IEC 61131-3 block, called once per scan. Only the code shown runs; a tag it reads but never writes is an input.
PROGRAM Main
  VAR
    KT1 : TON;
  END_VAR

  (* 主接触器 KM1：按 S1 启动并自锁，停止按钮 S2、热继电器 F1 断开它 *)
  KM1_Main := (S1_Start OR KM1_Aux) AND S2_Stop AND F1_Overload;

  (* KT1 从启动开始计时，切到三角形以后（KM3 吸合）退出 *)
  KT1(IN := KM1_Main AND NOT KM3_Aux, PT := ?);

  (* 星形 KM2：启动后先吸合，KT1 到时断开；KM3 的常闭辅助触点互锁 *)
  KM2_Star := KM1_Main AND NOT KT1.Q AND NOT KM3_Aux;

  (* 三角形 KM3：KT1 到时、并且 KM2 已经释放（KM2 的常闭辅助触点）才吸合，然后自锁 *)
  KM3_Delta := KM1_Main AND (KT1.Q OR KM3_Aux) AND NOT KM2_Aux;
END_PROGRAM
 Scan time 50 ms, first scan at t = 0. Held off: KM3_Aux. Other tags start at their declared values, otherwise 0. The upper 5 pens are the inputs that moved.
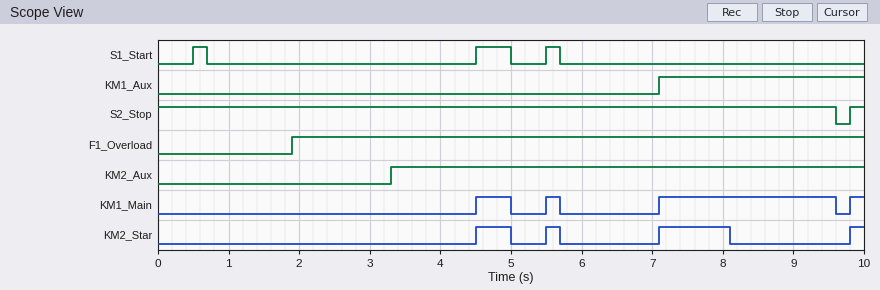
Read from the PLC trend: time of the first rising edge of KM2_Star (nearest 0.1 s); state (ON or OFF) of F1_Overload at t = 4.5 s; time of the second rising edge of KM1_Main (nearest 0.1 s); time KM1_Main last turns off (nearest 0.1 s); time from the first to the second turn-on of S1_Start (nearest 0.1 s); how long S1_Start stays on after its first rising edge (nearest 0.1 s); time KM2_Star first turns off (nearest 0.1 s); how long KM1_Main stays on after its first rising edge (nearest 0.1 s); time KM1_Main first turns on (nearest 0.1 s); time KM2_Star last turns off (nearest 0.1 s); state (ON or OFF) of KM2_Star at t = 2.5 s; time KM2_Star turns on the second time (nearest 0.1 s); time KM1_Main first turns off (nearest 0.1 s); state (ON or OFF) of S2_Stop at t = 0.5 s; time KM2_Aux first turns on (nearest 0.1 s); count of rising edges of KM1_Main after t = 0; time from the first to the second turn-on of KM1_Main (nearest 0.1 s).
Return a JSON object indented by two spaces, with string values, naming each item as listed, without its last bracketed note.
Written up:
{
  "time of the first rising edge of KM2_Star": "4.5 s",
  "state (ON or OFF) of F1_Overload at t = 4.5 s": "ON",
  "time of the second rising edge of KM1_Main": "5.5 s",
  "time KM1_Main last turns off": "9.6 s",
  "time from the first to the second turn-on of S1_Start": "4.0 s",
  "how long S1_Start stays on after its first rising edge": "0.2 s",
  "time KM2_Star first turns off": "5.0 s",
  "how long KM1_Main stays on after its first rising edge": "0.5 s",
  "time KM1_Main first turns on": "4.5 s",
  "time KM2_Star last turns off": "8.1 s",
  "state (ON or OFF) of KM2_Star at t = 2.5 s": "OFF",
  "time KM2_Star turns on the second time": "5.5 s",
  "time KM1_Main first turns off": "5.0 s",
  "state (ON or OFF) of S2_Stop at t = 0.5 s": "ON",
  "time KM2_Aux first turns on": "3.3 s",
  "count of rising edges of KM1_Main after t = 0": "4",
  "time from the first to the second turn-on of KM1_Main": "1.0 s"
}
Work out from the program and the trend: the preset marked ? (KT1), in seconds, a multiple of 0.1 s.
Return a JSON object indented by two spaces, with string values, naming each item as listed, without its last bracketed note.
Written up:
{
  "the preset marked ? (KT1), in seconds, a multiple of 0.1 s": "1.0 s"
}
